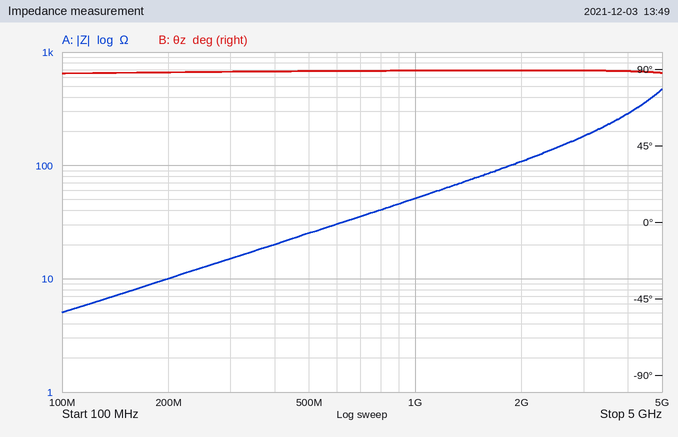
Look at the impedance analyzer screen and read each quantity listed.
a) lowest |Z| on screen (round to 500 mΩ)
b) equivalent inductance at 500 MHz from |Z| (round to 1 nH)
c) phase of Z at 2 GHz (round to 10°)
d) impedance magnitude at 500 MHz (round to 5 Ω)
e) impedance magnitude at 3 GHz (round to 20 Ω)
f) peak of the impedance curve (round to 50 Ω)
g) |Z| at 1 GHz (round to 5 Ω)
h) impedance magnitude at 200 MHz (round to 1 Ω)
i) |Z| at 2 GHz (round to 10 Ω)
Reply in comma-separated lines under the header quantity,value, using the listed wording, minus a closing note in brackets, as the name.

quantity,value
lowest |Z| on screen,5.0 Ω
equivalent inductance at 500 MHz from |Z|,8 nH
phase of Z at 2 GHz,90°
impedance magnitude at 500 MHz,25 Ω
impedance magnitude at 3 GHz,180 Ω
peak of the impedance curve,450 Ω
|Z| at 1 GHz,50 Ω
impedance magnitude at 200 MHz,10 Ω
|Z| at 2 GHz,110 Ω
